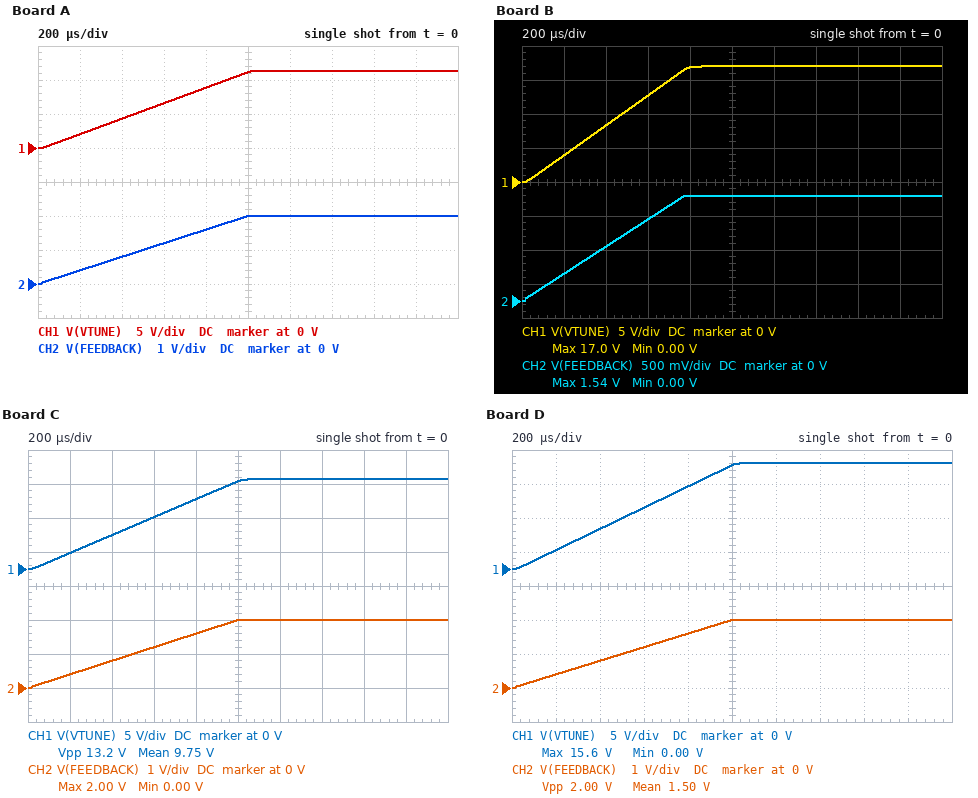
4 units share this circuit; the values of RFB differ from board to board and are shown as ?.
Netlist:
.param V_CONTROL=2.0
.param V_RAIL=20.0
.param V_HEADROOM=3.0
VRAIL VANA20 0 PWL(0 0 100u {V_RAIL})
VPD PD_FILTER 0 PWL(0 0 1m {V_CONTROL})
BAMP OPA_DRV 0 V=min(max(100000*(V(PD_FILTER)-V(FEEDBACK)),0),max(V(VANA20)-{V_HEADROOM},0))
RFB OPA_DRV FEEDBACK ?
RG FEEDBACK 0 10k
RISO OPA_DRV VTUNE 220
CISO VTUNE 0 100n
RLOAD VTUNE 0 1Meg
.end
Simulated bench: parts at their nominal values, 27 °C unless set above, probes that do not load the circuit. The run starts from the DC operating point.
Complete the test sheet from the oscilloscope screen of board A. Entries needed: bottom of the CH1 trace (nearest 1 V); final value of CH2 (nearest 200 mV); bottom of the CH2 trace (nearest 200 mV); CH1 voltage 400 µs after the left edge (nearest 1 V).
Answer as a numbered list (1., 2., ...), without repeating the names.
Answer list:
1. 0 V
2. 2.0 V
3. 0 V
4. 4 V
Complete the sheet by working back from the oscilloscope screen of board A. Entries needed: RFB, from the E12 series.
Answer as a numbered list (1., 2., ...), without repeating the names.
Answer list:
1. 47 kΩ
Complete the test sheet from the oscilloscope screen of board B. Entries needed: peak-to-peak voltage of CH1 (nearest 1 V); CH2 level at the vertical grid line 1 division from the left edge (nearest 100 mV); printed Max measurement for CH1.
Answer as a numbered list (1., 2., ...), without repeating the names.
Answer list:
1. 17 V
2. 400 mV
3. 17.0 V
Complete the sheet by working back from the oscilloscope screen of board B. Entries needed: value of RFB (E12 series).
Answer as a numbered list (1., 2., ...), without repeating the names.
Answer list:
1. 100 kΩ
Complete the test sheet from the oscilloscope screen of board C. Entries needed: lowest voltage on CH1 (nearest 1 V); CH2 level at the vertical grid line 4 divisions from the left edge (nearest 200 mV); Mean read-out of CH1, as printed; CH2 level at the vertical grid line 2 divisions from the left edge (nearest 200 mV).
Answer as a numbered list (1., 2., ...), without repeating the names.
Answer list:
1. 0 V
2. 1.6 V
3. 9.75 V
4. 800 mV
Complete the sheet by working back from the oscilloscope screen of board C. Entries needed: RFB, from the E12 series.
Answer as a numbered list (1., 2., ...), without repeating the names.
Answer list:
1. 56 kΩ
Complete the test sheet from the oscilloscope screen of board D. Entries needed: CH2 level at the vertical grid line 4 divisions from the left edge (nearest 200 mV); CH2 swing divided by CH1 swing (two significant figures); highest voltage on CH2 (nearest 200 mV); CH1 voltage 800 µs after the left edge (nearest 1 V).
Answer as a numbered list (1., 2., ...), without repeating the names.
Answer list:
1. 1.6 V
2. 0.13
3. 2.0 V
4. 12 V
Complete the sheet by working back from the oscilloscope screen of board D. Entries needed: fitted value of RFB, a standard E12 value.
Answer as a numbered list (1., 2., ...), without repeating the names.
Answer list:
1. 68 kΩ
